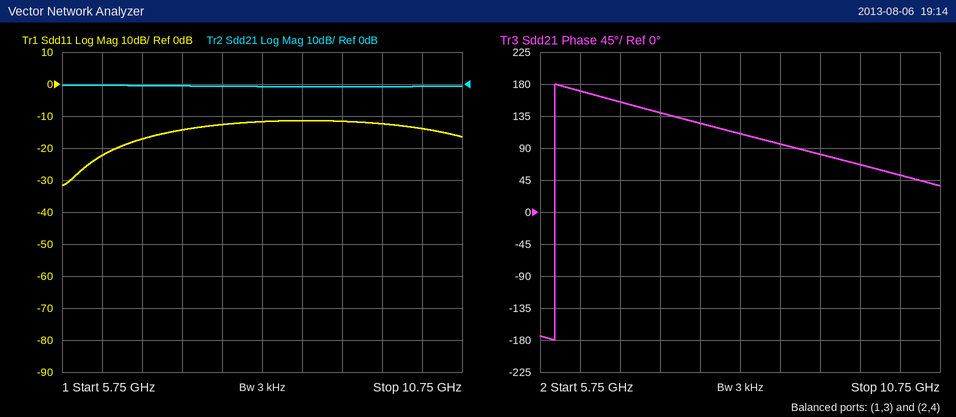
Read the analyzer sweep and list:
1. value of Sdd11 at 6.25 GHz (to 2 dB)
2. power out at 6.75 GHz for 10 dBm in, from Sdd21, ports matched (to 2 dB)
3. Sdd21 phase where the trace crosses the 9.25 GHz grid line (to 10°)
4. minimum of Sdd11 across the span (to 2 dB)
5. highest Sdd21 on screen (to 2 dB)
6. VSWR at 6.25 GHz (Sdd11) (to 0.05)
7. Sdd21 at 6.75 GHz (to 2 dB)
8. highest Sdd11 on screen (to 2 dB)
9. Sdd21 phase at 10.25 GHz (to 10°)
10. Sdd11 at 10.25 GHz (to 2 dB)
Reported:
-22 dB
10 dBm
80°
-32 dB
0 dB
1.15
0 dB
-12 dB
50°
-14 dB
